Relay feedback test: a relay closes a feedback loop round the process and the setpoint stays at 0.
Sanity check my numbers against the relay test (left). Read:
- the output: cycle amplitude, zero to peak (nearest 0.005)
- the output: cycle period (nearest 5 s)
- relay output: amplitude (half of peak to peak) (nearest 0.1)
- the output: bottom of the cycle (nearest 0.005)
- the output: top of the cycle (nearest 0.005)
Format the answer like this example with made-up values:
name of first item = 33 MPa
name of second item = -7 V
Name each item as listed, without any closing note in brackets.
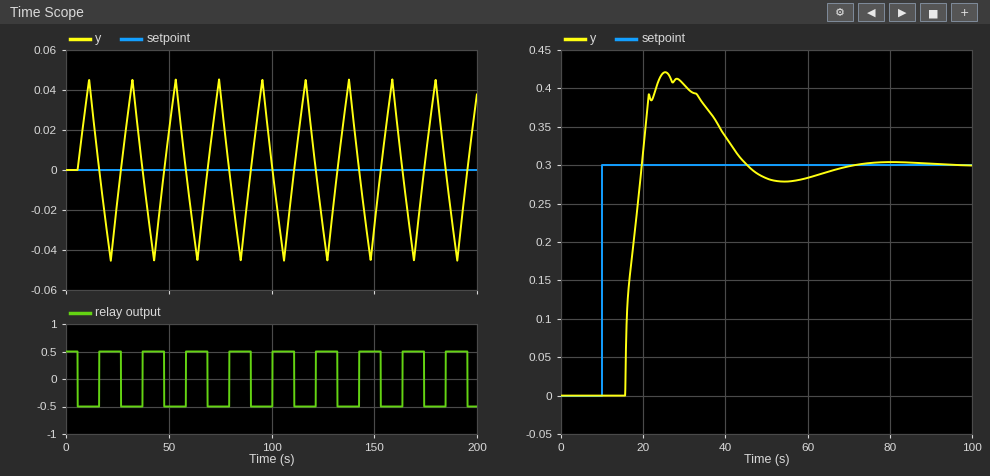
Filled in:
the output: cycle amplitude, zero to peak = 0.045
the output: cycle period = 20 s
relay output: amplitude (half of peak to peak) = 0.5
the output: bottom of the cycle = -0.045
the output: top of the cycle = 0.045
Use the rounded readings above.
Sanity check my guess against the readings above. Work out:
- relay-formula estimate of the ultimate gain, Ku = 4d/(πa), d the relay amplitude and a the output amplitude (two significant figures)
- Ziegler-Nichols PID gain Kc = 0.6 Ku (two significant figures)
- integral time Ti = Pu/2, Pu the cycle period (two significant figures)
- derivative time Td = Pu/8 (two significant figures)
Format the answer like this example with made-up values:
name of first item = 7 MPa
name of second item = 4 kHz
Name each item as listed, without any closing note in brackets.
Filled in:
relay-formula estimate of the ultimate gain, Ku = 4d/(πa), d the relay amplitude and a the output amplitude = 14
Ziegler-Nichols PID gain Kc = 0.6 Ku = 8.4
integral time Ti = Pu/2, Pu the cycle period = 10 s
derivative time Td = Pu/8 = 2.5 s
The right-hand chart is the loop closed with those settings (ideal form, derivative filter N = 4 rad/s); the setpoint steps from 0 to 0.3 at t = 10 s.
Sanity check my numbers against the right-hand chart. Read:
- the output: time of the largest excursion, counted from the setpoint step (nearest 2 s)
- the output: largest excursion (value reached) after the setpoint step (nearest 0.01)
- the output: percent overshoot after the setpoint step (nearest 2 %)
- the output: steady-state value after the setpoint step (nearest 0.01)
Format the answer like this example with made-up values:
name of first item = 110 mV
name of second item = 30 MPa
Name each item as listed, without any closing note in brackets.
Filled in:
the output: time of the largest excursion, counted from the setpoint step = 16 s
the output: largest excursion (value reached) after the setpoint step = 0.42
the output: percent overshoot after the setpoint step = 40 %
the output: steady-state value after the setpoint step = 0.30
